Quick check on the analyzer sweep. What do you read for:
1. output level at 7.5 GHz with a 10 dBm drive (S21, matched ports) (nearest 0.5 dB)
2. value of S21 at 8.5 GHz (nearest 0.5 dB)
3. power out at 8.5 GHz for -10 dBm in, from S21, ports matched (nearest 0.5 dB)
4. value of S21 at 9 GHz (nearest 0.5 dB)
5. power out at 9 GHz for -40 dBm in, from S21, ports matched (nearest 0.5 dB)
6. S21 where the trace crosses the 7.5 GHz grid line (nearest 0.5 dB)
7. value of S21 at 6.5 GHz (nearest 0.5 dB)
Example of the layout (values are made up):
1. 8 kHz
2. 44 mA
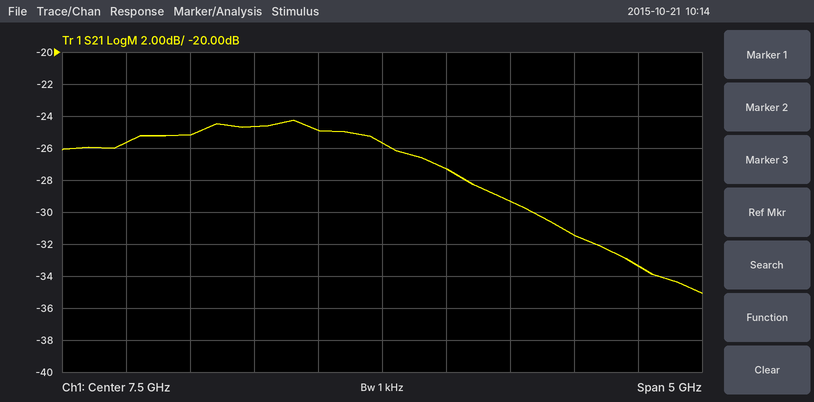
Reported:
1. -15.5 dBm
2. -29.5 dB
3. -39.5 dBm
4. -31.5 dB
5. -71.5 dBm
6. -25.5 dB
7. -24.5 dB
